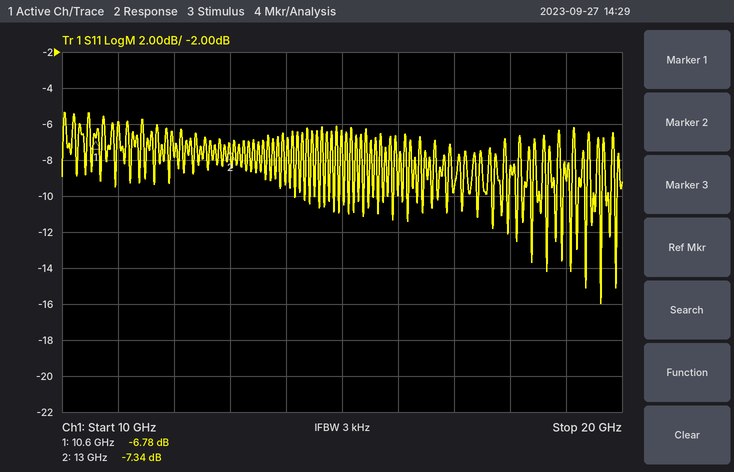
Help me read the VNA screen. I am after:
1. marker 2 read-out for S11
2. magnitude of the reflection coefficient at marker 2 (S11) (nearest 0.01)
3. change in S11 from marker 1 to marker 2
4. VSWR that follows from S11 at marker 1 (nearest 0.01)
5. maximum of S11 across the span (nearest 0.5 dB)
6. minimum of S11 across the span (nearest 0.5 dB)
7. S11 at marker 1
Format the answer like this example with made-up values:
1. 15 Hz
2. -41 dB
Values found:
1. -7.34 dB
2. 0.43
3. -0.56 dB
4. 2.69
5. -5.5 dB
6. -16.0 dB
7. -6.78 dB
